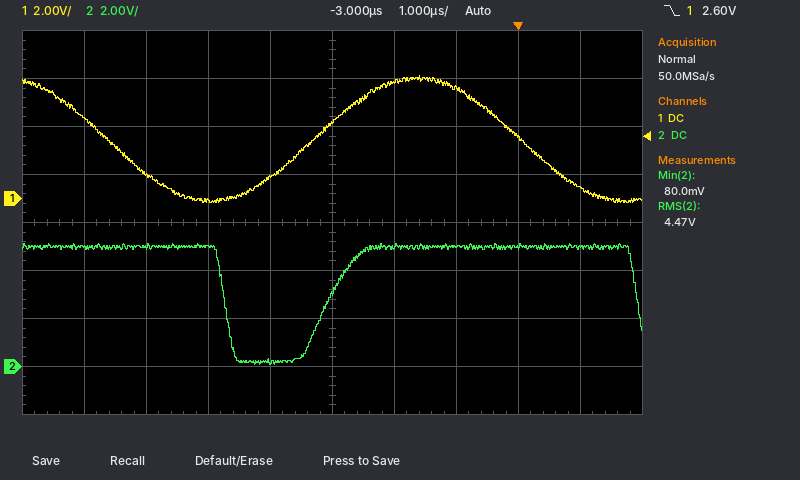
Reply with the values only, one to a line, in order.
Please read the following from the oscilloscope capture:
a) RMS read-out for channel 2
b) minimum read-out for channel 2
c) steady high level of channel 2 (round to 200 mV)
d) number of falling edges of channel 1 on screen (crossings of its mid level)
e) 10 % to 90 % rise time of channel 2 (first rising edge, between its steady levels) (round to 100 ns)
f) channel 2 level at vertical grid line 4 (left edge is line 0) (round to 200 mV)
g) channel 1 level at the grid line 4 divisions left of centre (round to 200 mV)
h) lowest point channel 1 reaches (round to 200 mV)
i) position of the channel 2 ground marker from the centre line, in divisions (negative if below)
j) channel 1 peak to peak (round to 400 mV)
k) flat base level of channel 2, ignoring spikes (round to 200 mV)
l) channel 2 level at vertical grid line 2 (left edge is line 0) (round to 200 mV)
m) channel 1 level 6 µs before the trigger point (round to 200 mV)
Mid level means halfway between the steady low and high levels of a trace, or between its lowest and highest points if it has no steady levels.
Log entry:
4.47 V
80.0 mV
5.0 V
2
800 ns
200 mV
3.4 V
-200 mV
-3.0 div
5.2 V
200 mV
5.0 V
1.0 V
